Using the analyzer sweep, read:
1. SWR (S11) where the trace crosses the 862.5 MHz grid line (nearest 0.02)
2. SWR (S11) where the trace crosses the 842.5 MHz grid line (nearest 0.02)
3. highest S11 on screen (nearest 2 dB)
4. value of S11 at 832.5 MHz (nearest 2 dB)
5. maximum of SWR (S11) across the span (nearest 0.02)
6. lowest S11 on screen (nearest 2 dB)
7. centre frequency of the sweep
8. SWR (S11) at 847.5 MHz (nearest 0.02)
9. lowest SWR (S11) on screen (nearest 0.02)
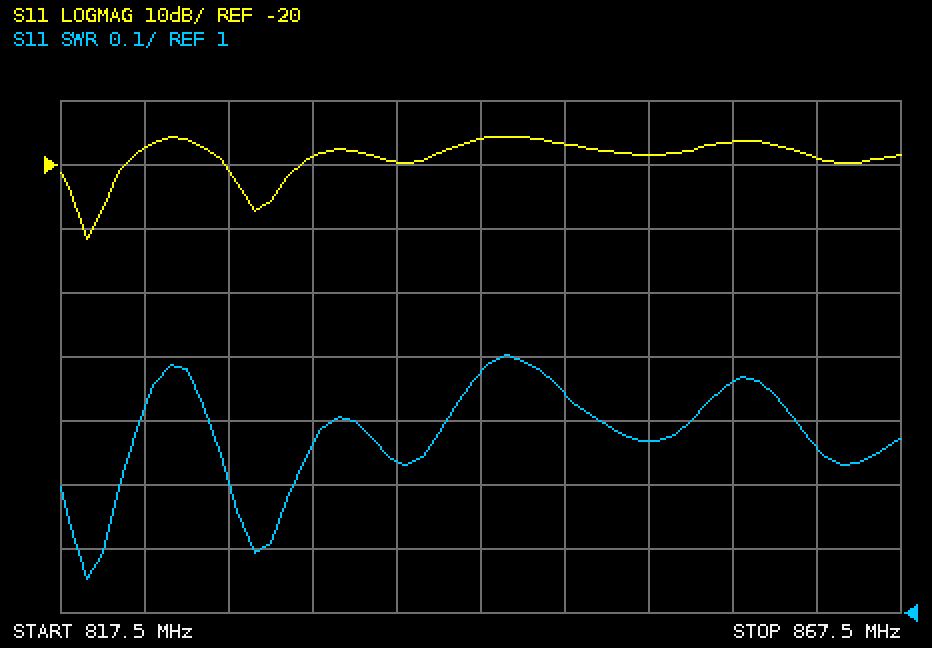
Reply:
1.26
1.38
-16 dB
-18 dB
1.40
-32 dB
842.5 MHz
1.34
1.06
